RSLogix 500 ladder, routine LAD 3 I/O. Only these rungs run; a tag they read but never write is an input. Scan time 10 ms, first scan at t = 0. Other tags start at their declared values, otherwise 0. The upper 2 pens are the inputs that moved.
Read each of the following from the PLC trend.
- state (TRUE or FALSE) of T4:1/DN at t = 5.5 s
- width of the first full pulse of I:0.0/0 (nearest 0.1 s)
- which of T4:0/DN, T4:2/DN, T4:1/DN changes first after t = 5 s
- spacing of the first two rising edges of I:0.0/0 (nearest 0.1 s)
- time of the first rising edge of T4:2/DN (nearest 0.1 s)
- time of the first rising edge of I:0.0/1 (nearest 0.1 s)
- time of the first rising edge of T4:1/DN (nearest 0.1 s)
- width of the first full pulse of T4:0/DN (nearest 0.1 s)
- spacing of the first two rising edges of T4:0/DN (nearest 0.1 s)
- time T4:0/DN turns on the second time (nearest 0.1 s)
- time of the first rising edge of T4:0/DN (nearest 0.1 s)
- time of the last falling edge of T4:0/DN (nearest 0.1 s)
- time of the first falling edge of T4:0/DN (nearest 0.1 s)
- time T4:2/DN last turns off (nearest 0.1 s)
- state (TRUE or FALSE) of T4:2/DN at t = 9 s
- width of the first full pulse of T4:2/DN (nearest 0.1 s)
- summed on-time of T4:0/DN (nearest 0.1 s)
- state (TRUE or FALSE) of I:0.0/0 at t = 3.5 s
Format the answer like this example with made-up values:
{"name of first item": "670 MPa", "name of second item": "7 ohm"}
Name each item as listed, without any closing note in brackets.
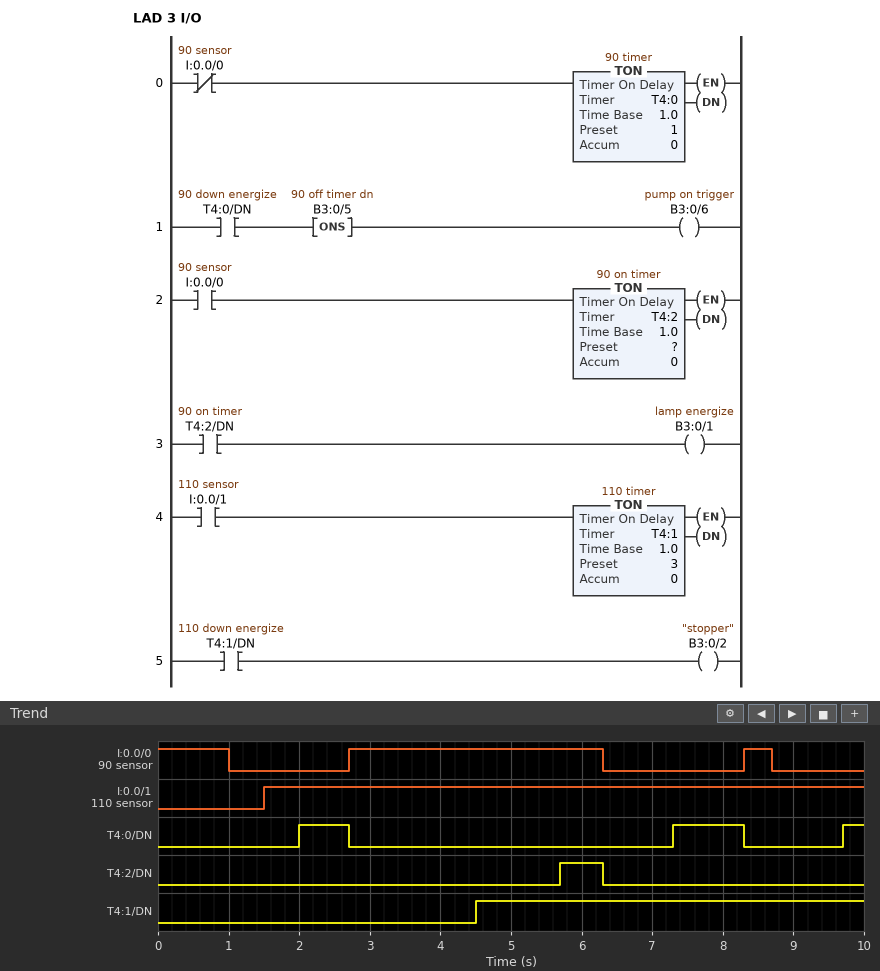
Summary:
{"state (TRUE or FALSE) of T4:1/DN at t = 5.5 s": "TRUE", "width of the first full pulse of I:0.0/0": "3.6 s", "which of T4:0/DN, T4:2/DN, T4:1/DN changes first after t = 5 s": "T4:2/DN", "spacing of the first two rising edges of I:0.0/0": "5.6 s", "time of the first rising edge of T4:2/DN": "5.7 s", "time of the first rising edge of I:0.0/1": "1.5 s", "time of the first rising edge of T4:1/DN": "4.5 s", "width of the first full pulse of T4:0/DN": "0.7 s", "spacing of the first two rising edges of T4:0/DN": "5.3 s", "time T4:0/DN turns on the second time": "7.3 s", "time of the first rising edge of T4:0/DN": "2.0 s", "time of the last falling edge of T4:0/DN": "8.3 s", "time of the first falling edge of T4:0/DN": "2.7 s", "time T4:2/DN last turns off": "6.3 s", "state (TRUE or FALSE) of T4:2/DN at t = 9 s": "FALSE", "width of the first full pulse of T4:2/DN": "0.6 s", "summed on-time of T4:0/DN": "2.0 s", "state (TRUE or FALSE) of I:0.0/0 at t = 3.5 s": "TRUE"}
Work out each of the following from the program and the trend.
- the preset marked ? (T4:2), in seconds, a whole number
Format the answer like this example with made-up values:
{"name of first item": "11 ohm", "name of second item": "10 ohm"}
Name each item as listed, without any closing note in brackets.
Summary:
{"the preset marked ? (T4:2), in seconds, a whole number": "3 s"}
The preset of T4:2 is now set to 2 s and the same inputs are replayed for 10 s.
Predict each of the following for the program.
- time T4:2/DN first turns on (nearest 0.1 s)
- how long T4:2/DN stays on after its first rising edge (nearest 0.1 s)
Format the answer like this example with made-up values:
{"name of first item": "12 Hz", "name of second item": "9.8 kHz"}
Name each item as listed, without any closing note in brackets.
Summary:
{"time T4:2/DN first turns on": "4.7 s", "how long T4:2/DN stays on after its first rising edge": "1.6 s"}
